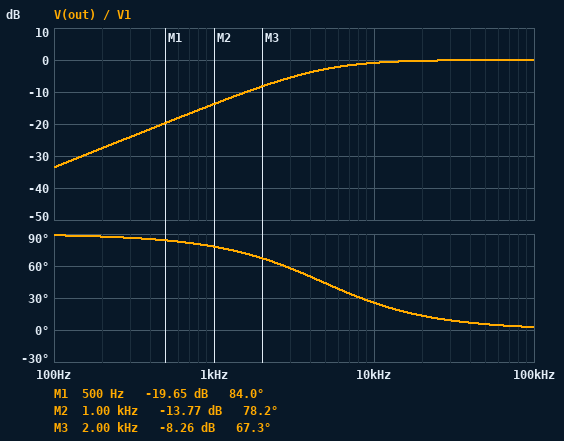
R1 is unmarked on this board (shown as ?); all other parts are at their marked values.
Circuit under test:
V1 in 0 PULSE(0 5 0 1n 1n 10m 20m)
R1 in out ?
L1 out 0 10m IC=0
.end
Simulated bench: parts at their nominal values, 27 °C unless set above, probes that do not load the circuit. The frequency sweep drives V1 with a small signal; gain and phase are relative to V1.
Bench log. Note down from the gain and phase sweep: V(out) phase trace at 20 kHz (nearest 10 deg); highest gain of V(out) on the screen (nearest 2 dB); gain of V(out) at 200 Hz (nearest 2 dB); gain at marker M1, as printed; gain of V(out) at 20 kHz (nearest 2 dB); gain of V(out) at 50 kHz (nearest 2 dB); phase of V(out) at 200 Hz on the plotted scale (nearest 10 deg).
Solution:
10 deg
0 dB
-28 dB
-19.65 dB
0 dB
0 dB
90 deg
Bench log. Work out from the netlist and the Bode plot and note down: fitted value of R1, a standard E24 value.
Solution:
300 Ω
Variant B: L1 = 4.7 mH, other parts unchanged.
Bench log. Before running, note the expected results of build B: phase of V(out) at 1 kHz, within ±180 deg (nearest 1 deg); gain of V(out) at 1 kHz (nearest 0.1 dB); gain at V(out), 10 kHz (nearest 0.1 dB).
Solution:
84 deg
-20.2 dB
-3.1 dB
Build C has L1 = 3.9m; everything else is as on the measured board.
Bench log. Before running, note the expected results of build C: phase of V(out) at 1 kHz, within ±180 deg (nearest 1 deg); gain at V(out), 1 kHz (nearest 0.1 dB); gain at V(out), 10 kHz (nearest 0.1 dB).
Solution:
85 deg
-21.8 dB
-4.0 dB
